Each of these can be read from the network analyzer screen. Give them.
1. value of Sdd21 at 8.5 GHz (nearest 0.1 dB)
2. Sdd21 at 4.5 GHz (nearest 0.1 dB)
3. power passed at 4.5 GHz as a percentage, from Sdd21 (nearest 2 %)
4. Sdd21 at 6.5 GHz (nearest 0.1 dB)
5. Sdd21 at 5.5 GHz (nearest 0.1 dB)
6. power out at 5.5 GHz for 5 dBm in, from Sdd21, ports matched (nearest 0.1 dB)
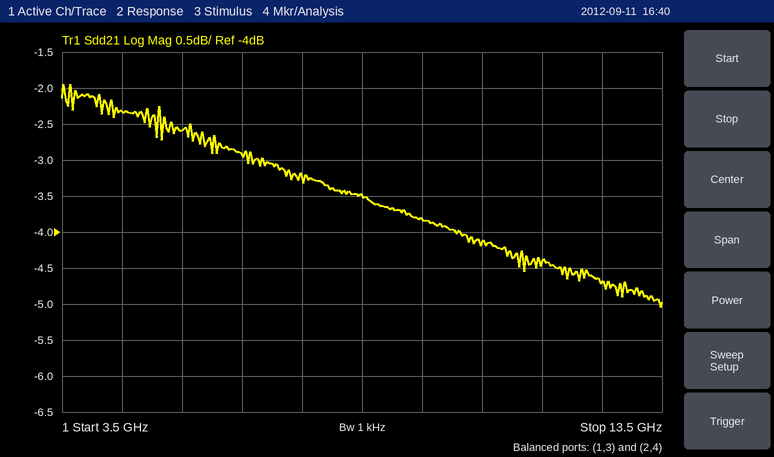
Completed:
-3.5 dB
-2.3 dB
58 %
-2.9 dB
-2.6 dB
2.4 dBm
